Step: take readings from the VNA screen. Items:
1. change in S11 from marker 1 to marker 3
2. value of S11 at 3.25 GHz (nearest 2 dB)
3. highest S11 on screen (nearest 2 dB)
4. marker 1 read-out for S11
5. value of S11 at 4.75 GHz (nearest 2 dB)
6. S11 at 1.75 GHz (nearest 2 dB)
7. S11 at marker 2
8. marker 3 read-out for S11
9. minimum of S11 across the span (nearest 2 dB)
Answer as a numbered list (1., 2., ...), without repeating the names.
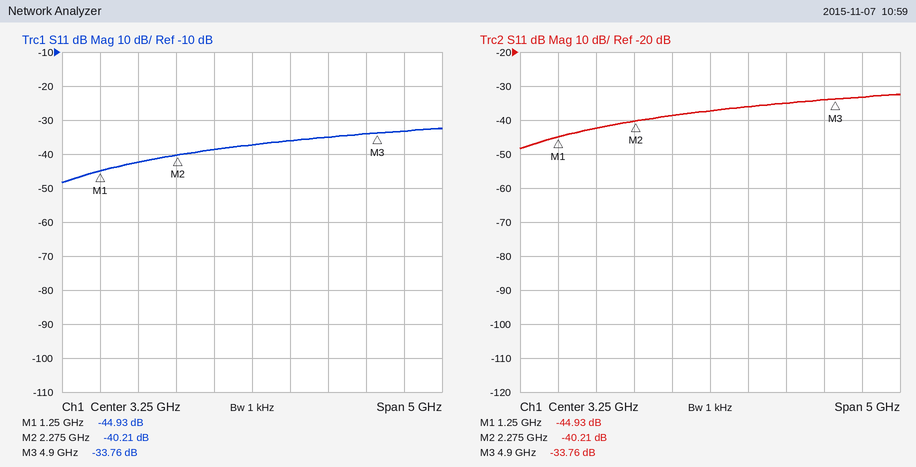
1. 11.17 dB
2. -38 dB
3. -32 dB
4. -44.93 dB
5. -34 dB
6. -42 dB
7. -40.21 dB
8. -33.76 dB
9. -48 dB
